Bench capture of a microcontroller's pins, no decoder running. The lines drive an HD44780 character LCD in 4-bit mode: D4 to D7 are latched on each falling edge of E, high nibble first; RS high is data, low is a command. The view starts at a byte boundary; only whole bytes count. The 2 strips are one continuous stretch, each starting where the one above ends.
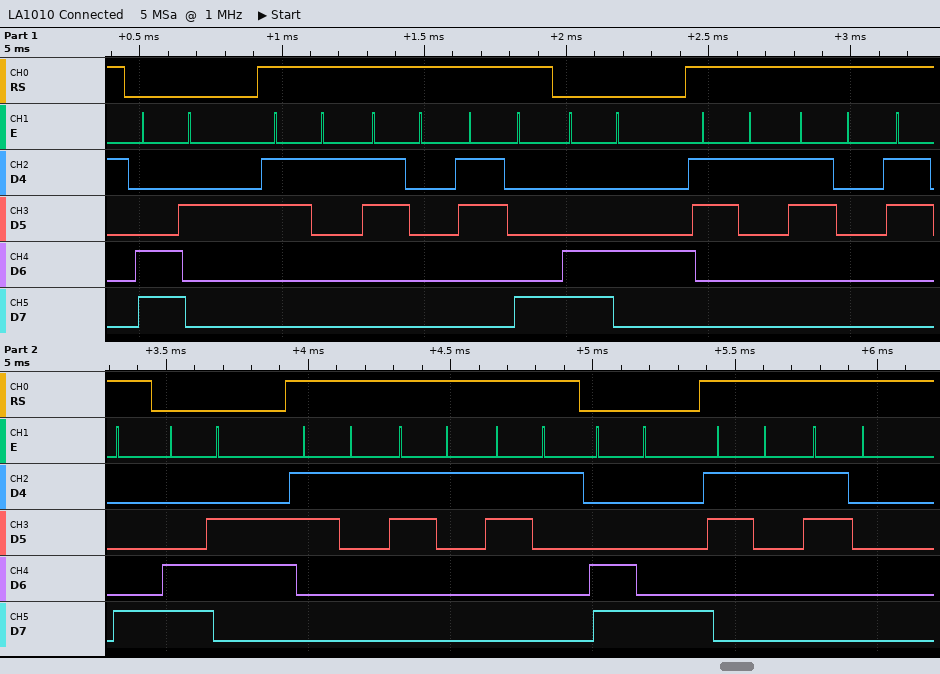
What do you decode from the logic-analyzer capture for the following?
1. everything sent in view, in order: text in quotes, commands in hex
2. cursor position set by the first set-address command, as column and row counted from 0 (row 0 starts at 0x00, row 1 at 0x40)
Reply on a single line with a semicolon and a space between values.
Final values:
0xC2 "108" 0xC4 "108" 0xC6 "111" 0xC8 "10"; column 2, row 1
